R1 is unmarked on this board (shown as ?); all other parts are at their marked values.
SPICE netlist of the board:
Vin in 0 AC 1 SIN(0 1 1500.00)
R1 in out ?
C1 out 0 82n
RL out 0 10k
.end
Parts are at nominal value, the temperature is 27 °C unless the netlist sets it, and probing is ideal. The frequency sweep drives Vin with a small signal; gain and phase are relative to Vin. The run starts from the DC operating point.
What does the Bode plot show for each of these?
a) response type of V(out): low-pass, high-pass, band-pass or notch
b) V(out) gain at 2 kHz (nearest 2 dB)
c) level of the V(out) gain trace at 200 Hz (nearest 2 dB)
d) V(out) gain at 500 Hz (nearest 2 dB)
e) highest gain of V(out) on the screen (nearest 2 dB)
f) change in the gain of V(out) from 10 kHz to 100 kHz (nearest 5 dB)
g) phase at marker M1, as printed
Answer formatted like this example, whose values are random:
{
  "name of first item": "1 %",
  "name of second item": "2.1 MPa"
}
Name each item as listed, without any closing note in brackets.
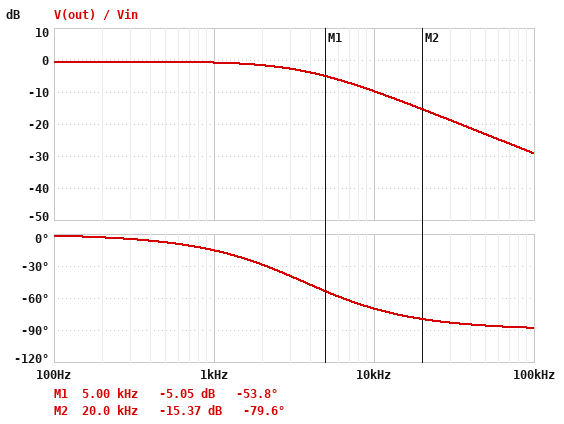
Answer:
{
  "response type of V(out): low-pass, high-pass, band-pass or notch": "low-pass",
  "V(out) gain at 2 kHz": "-2 dB",
  "level of the V(out) gain trace at 200 Hz": "0 dB",
  "V(out) gain at 500 Hz": "0 dB",
  "highest gain of V(out) on the screen": "0 dB",
  "change in the gain of V(out) from 10 kHz to 100 kHz": "-20 dB",
  "phase at marker M1, as printed": "-53.8 deg"
}
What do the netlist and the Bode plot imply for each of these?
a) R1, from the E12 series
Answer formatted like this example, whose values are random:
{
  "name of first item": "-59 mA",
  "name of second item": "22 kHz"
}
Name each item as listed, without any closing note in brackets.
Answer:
{
  "R1, from the E12 series": "560 Ω"
}
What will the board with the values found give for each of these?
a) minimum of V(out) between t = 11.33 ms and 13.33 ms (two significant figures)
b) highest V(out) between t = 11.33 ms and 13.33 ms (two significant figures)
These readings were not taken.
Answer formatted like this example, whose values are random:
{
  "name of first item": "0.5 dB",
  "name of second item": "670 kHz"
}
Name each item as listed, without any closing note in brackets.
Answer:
{
  "minimum of V(out) between t = 11.33 ms and 13.33 ms": "-880 mV",
  "highest V(out) between t = 11.33 ms and 13.33 ms": "880 mV"
}
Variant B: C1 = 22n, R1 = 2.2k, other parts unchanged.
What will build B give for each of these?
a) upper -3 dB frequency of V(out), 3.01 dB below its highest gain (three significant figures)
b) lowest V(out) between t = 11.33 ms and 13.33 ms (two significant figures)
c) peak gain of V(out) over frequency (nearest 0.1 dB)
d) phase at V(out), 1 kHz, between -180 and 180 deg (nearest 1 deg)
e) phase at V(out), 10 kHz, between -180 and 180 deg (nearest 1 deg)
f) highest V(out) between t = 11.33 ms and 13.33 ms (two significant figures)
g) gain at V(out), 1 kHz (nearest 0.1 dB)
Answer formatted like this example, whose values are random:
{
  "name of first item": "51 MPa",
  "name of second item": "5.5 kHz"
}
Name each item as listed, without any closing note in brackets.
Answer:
{
  "upper -3 dB frequency of V(out), 3.01 dB below its highest gain": "4.01 kHz",
  "lowest V(out) between t = 11.33 ms and 13.33 ms": "-770 mV",
  "peak gain of V(out) over frequency": "-1.7 dB",
  "phase at V(out), 1 kHz, between -180 and 180 deg": "-14 deg",
  "phase at V(out), 10 kHz, between -180 and 180 deg": "-68 deg",
  "highest V(out) between t = 11.33 ms and 13.33 ms": "770 mV",
  "gain at V(out), 1 kHz": "-2.0 dB"
}
